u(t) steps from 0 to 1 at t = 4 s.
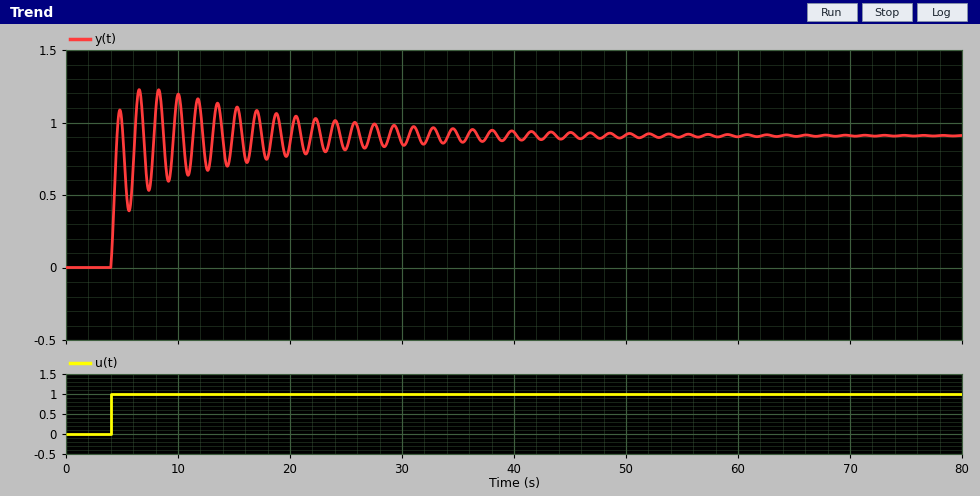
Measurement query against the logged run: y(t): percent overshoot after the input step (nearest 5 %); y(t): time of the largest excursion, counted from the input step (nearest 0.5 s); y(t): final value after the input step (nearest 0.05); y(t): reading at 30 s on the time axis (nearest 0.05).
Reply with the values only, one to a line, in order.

35 %
2.5 s
0.90
0.85
